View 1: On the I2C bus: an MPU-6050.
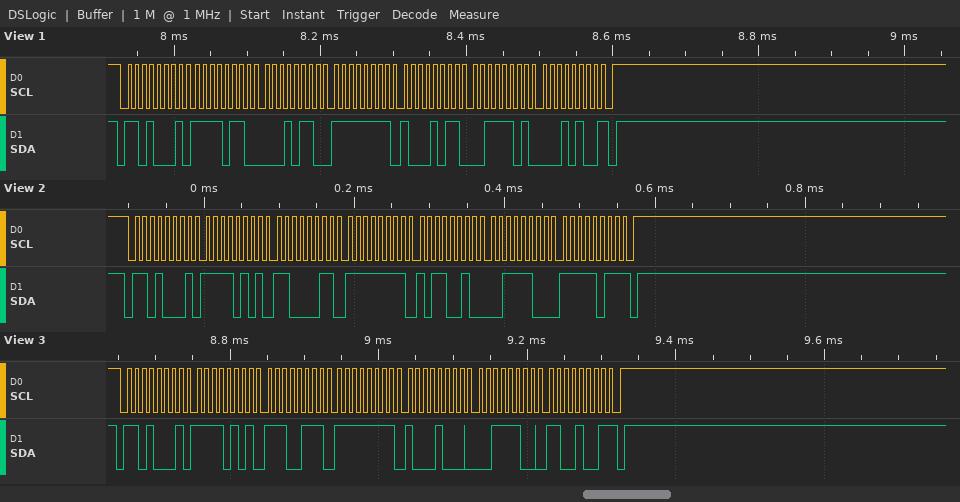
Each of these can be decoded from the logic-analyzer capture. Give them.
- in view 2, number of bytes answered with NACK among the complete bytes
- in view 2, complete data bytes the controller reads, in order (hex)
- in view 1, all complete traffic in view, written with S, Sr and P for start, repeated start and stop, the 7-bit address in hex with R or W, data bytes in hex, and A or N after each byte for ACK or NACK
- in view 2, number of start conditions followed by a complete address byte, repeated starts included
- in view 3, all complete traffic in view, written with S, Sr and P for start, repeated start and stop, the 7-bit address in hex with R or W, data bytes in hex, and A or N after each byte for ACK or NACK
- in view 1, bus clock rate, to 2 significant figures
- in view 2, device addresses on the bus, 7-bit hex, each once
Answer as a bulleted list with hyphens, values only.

- 1
- F5 C3 FF B2 3C FB
- S 68R A F6 A 16 A FF A 8B A 3D A 14 N P
- 1
- S 68R A F5 A E7 A FF A 88 A 3C A C9 N P
- 100 kHz
- 0x68
